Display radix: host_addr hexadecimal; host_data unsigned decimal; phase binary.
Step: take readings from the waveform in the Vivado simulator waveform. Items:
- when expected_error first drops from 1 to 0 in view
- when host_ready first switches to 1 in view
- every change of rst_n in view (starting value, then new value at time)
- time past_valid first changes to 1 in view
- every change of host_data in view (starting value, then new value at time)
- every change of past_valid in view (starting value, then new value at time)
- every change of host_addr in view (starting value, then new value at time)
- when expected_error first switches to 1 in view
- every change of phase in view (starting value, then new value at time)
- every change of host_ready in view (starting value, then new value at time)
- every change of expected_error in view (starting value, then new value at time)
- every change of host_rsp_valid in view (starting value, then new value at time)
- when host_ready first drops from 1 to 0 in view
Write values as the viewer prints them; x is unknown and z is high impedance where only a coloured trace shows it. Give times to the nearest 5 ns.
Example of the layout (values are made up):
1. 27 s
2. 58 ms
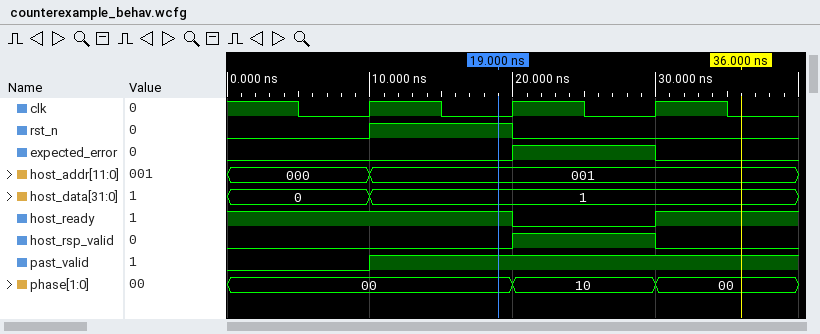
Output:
1. 30 ns
2. 30 ns
3. 0, 1 at 10 ns, 0 at 20 ns
4. 10 ns
5. 0, 1 at 10 ns
6. 0, 1 at 10 ns
7. 000, 001 at 10 ns
8. 20 ns
9. 00, 10 at 20 ns, 00 at 30 ns
10. 1, 0 at 20 ns, 1 at 30 ns
11. 0, 1 at 20 ns, 0 at 30 ns
12. 0, 1 at 20 ns, 0 at 30 ns
13. 20 ns
